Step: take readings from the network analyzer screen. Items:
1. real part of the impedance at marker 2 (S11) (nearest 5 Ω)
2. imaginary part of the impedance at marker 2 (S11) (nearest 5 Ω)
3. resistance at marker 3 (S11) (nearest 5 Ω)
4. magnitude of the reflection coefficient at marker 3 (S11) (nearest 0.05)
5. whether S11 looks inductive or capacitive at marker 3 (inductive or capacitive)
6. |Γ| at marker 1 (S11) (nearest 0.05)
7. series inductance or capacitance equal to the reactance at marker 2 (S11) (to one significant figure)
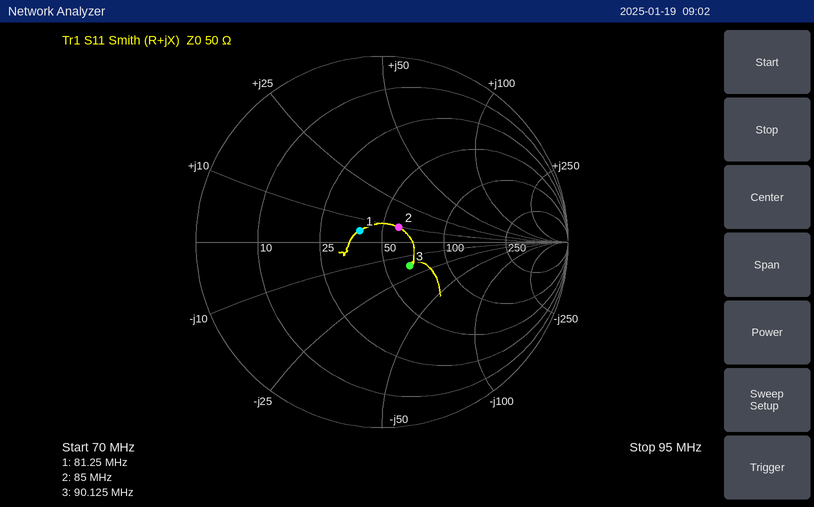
60 Ω
+10 Ω
65 Ω
0.20
capacitive
0.15
20 nH
